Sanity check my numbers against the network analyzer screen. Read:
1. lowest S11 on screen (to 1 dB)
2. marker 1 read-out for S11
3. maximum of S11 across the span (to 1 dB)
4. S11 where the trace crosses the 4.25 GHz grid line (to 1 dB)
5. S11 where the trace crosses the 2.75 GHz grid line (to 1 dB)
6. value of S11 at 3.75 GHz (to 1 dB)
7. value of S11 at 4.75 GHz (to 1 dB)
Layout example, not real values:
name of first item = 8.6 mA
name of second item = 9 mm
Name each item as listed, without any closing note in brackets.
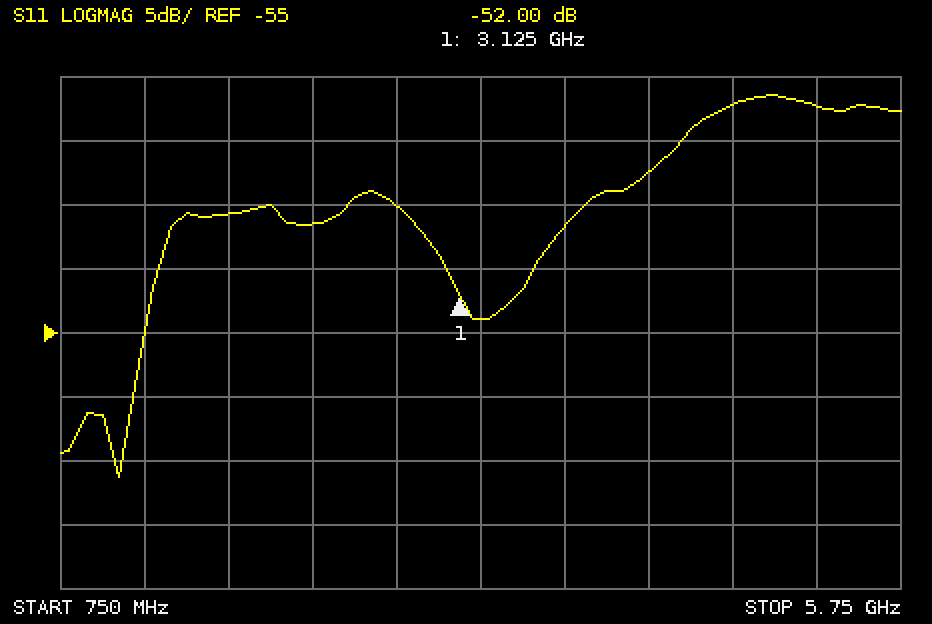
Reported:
lowest S11 on screen = -66 dB
marker 1 read-out for S11 = -52.00 dB
maximum of S11 across the span = -36 dB
S11 where the trace crosses the 4.25 GHz grid line = -42 dB
S11 where the trace crosses the 2.75 GHz grid line = -45 dB
value of S11 at 3.75 GHz = -47 dB
value of S11 at 4.75 GHz = -37 dB
